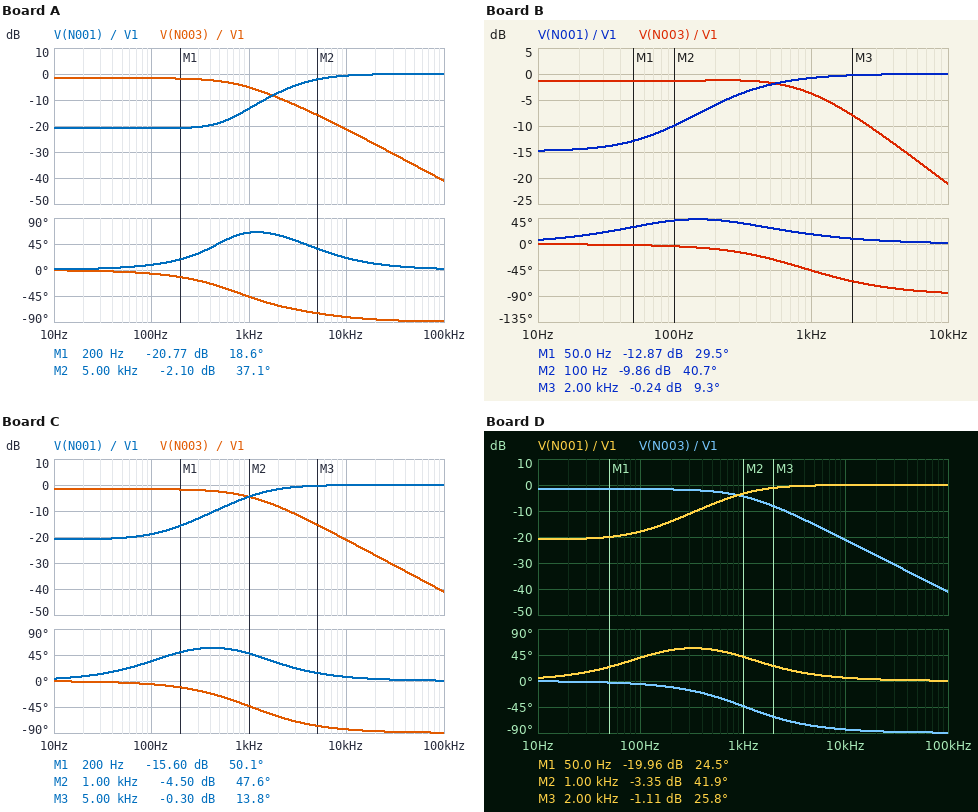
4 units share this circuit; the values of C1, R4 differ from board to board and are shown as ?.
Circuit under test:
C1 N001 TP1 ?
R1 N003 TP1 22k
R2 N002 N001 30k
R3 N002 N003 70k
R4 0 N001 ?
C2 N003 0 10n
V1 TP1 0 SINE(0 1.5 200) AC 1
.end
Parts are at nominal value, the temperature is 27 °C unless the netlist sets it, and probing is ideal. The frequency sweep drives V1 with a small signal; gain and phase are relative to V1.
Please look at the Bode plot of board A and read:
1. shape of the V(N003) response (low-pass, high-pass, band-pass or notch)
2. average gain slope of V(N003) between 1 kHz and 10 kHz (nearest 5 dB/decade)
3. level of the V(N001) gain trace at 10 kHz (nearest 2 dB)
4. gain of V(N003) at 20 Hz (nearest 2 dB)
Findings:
low-pass
-15 dB/decade
0 dB
-2 dB
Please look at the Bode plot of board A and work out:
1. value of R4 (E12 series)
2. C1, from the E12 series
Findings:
12 kΩ
3.9 nF
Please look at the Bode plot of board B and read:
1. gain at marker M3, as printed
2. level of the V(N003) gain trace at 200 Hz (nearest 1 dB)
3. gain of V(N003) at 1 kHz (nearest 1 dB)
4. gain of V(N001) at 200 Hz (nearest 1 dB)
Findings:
-0.24 dB
-1 dB
-4 dB
-6 dB
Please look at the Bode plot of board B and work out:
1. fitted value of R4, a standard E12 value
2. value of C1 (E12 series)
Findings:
27 kΩ
22 nF
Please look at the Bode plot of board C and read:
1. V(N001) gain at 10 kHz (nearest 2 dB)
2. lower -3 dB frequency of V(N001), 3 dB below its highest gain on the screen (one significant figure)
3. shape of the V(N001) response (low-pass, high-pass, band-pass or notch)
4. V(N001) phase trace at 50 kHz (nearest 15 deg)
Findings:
0 dB
1 kHz
high-pass
0 deg
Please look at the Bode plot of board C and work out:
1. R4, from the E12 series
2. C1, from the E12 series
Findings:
12 kΩ
12 nF
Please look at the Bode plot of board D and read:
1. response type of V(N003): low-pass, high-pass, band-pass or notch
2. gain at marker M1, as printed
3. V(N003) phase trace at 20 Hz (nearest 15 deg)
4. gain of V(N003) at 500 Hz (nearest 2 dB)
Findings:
low-pass
-19.96 dB
0 deg
-2 dB
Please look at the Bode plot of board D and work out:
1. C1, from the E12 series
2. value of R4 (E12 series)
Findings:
15 nF
12 kΩ
